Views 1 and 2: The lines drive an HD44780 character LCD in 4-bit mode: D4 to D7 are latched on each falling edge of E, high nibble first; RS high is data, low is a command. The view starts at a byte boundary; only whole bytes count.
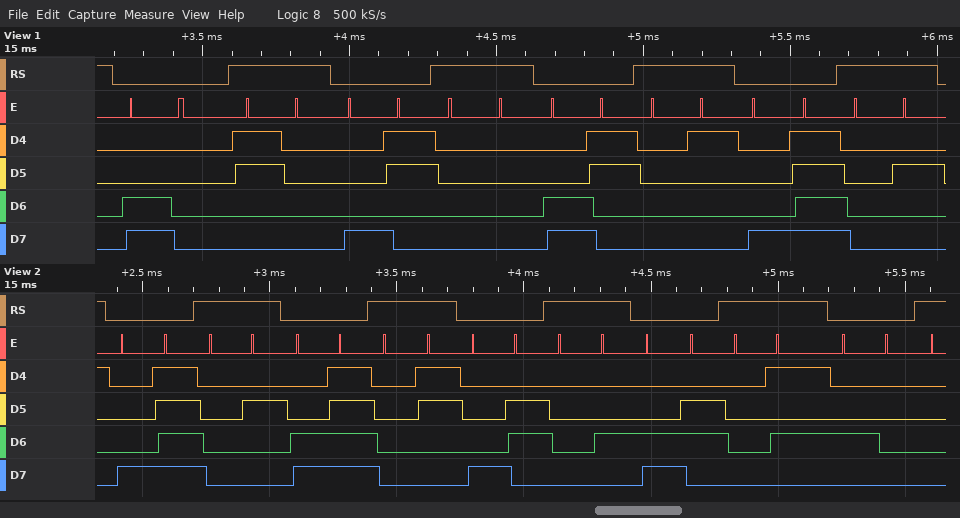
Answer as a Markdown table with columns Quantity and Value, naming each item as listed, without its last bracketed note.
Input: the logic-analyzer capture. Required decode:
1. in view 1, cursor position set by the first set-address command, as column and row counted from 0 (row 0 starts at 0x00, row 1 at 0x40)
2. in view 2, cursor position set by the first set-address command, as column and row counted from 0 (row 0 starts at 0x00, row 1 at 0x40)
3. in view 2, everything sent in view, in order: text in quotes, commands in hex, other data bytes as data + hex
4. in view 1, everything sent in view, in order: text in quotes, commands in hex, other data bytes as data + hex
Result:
| Quantity | Value |
|---|---|
| in view 1, cursor position set by the first set-address command, as column and row counted from 0 | column 0, row 1 |
| in view 2, cursor position set by the first set-address command, as column and row counted from 0 | column 15, row 0 |
| in view 2, everything sent in view, in order: text in quotes, commands in hex, other data bytes as data + hex | 0x8F data 02 0xCF data 03 0x86 data 04 0xC6 data 05 0x40 |
| in view 1, everything sent in view, in order: text in quotes, commands in hex, other data bytes as data + hex | 0xC0 "0" 0x83 data 00 0xC3 data 01 0x8F data 02 |
